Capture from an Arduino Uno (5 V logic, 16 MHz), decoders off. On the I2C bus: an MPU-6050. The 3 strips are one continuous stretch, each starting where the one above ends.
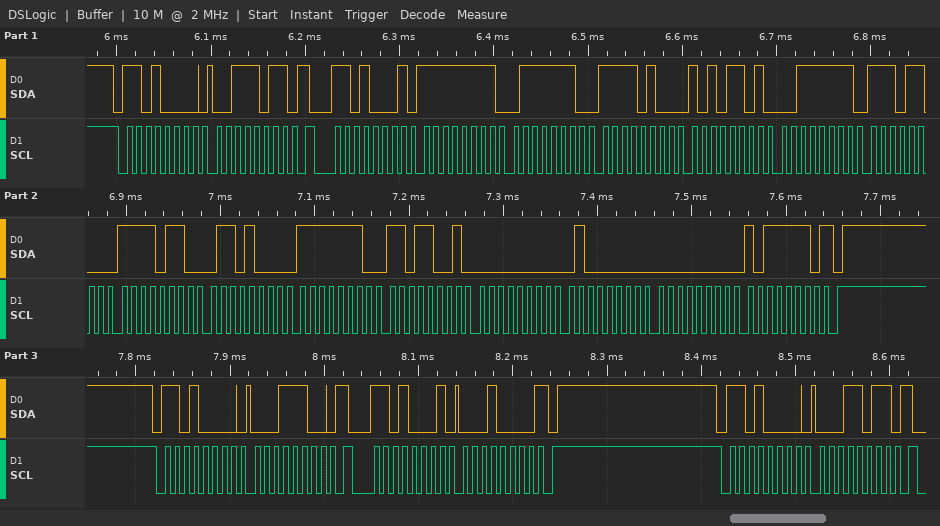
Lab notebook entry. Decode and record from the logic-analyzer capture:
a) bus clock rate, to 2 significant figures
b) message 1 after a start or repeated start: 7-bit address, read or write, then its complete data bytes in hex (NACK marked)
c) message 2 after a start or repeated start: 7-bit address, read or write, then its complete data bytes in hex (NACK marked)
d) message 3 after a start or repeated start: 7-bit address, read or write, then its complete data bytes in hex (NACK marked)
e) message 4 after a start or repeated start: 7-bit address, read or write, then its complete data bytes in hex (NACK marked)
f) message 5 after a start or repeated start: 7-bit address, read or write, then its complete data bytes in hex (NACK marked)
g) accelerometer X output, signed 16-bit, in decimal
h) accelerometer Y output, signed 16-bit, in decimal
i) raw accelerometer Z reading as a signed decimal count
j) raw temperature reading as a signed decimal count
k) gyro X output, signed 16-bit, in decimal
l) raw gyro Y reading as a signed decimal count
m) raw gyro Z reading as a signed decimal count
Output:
100 kHz
0x68 write: 3B
0x68 read: FF 7E F4 AD 3F EC F6 68 FE D9 00 40 00 BE NACK
0x68 write: 1C
0x68 read: 10 NACK
0x68 write: 1B
-130
-2899
16364
-2456
-295
64
190
